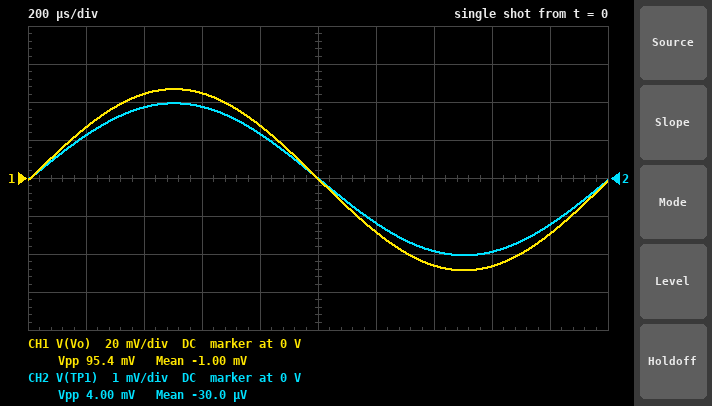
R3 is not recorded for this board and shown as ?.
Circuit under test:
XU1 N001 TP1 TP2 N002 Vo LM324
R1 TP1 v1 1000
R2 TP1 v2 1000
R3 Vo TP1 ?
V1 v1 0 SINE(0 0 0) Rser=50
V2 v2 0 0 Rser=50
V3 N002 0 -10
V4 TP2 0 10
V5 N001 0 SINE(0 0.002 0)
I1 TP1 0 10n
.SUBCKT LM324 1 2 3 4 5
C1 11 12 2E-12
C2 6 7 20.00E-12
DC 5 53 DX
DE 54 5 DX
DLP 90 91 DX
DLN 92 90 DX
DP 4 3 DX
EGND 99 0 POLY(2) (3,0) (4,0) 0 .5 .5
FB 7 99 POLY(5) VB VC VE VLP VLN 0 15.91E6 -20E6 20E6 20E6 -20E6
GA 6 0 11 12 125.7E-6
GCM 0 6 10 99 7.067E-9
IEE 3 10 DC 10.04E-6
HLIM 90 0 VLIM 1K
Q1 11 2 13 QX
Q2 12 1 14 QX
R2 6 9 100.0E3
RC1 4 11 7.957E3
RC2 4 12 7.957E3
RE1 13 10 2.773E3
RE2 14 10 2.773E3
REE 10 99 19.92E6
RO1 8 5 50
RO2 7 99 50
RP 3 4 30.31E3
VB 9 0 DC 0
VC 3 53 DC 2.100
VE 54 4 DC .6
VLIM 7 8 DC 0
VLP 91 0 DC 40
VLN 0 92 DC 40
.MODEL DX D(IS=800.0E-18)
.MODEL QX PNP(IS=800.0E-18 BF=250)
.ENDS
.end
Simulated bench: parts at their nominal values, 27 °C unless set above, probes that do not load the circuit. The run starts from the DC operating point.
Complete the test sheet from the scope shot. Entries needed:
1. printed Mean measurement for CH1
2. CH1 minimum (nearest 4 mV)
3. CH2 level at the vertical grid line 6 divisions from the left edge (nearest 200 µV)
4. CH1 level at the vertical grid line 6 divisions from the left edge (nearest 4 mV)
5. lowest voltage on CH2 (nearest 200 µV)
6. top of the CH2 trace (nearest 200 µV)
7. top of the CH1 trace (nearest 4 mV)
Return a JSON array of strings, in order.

["-1.00 mV", "-48 mV", "-1.2 mV", "-28 mV", "-2.0 mV", "2.0 mV", "48 mV"]
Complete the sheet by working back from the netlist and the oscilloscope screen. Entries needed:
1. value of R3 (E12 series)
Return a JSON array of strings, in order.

["12 kΩ"]
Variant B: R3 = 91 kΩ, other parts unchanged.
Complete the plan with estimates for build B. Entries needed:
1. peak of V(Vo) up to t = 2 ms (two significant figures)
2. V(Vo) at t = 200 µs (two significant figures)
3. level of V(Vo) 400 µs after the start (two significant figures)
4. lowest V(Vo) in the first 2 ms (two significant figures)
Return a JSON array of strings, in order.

["340 mV", "170 mV", "310 mV", "-350 mV"]
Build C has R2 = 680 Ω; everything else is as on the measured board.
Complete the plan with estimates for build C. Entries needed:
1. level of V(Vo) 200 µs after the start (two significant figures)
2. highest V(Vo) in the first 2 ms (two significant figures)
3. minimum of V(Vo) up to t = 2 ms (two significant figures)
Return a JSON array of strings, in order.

["32 mV", "57 mV", "-59 mV"]
